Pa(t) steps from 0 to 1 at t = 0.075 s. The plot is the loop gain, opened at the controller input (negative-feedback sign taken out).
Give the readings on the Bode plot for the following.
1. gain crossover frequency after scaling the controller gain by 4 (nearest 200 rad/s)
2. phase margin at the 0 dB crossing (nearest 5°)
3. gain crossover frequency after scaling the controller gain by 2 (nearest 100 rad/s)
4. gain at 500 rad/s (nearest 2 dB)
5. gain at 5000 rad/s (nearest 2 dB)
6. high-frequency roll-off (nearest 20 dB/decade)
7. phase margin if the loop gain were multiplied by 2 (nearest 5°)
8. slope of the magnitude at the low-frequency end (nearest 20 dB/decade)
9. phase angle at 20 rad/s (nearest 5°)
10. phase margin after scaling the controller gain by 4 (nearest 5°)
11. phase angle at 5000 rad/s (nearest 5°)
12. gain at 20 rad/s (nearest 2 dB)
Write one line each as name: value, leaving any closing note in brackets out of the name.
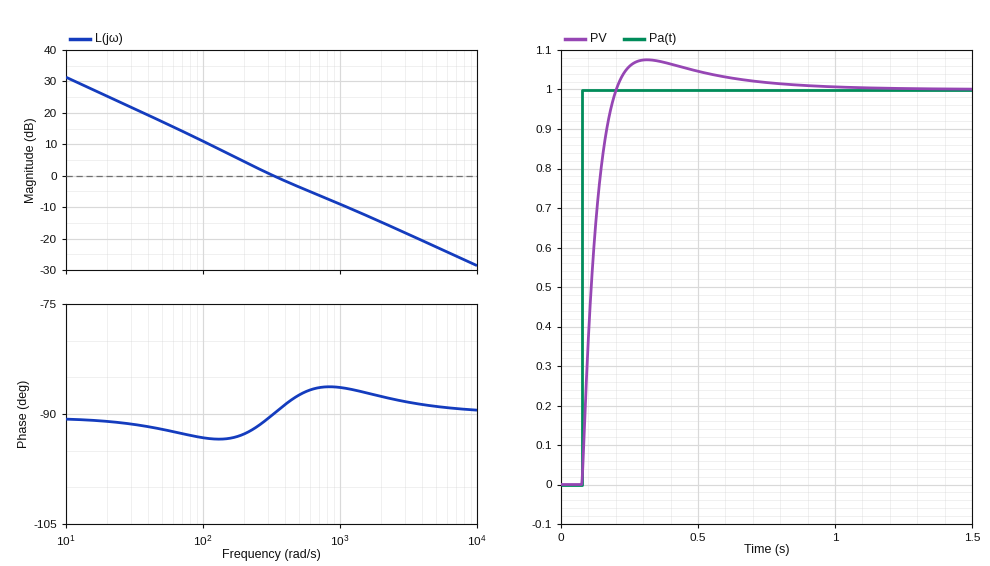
gain crossover frequency after scaling the controller gain by 4: 1400 rad/s
phase margin at the 0 dB crossing: 90°
gain crossover frequency after scaling the controller gain by 2: 700 rad/s
gain at 500 rad/s: -4 dB
gain at 5000 rad/s: -22 dB
high-frequency roll-off: -20 dB/decade
phase margin if the loop gain were multiplied by 2: 95°
slope of the magnitude at the low-frequency end: -20 dB/decade
phase angle at 20 rad/s: -90°
phase margin after scaling the controller gain by 4: 95°
phase angle at 5000 rad/s: -90°
gain at 20 rad/s: 26 dB
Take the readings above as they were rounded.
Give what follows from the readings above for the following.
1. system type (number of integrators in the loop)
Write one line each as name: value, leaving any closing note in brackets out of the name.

system type: 1
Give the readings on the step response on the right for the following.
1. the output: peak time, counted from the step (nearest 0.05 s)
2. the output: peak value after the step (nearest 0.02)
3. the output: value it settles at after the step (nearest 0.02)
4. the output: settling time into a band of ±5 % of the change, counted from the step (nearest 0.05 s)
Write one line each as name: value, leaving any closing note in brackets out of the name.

the output: peak time, counted from the step: 0.25 s
the output: peak value after the step: 1.08
the output: value it settles at after the step: 1.00
the output: settling time into a band of ±5 % of the change, counted from the step: 0.40 s
